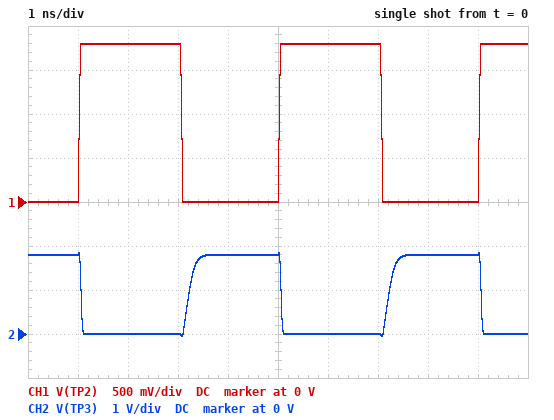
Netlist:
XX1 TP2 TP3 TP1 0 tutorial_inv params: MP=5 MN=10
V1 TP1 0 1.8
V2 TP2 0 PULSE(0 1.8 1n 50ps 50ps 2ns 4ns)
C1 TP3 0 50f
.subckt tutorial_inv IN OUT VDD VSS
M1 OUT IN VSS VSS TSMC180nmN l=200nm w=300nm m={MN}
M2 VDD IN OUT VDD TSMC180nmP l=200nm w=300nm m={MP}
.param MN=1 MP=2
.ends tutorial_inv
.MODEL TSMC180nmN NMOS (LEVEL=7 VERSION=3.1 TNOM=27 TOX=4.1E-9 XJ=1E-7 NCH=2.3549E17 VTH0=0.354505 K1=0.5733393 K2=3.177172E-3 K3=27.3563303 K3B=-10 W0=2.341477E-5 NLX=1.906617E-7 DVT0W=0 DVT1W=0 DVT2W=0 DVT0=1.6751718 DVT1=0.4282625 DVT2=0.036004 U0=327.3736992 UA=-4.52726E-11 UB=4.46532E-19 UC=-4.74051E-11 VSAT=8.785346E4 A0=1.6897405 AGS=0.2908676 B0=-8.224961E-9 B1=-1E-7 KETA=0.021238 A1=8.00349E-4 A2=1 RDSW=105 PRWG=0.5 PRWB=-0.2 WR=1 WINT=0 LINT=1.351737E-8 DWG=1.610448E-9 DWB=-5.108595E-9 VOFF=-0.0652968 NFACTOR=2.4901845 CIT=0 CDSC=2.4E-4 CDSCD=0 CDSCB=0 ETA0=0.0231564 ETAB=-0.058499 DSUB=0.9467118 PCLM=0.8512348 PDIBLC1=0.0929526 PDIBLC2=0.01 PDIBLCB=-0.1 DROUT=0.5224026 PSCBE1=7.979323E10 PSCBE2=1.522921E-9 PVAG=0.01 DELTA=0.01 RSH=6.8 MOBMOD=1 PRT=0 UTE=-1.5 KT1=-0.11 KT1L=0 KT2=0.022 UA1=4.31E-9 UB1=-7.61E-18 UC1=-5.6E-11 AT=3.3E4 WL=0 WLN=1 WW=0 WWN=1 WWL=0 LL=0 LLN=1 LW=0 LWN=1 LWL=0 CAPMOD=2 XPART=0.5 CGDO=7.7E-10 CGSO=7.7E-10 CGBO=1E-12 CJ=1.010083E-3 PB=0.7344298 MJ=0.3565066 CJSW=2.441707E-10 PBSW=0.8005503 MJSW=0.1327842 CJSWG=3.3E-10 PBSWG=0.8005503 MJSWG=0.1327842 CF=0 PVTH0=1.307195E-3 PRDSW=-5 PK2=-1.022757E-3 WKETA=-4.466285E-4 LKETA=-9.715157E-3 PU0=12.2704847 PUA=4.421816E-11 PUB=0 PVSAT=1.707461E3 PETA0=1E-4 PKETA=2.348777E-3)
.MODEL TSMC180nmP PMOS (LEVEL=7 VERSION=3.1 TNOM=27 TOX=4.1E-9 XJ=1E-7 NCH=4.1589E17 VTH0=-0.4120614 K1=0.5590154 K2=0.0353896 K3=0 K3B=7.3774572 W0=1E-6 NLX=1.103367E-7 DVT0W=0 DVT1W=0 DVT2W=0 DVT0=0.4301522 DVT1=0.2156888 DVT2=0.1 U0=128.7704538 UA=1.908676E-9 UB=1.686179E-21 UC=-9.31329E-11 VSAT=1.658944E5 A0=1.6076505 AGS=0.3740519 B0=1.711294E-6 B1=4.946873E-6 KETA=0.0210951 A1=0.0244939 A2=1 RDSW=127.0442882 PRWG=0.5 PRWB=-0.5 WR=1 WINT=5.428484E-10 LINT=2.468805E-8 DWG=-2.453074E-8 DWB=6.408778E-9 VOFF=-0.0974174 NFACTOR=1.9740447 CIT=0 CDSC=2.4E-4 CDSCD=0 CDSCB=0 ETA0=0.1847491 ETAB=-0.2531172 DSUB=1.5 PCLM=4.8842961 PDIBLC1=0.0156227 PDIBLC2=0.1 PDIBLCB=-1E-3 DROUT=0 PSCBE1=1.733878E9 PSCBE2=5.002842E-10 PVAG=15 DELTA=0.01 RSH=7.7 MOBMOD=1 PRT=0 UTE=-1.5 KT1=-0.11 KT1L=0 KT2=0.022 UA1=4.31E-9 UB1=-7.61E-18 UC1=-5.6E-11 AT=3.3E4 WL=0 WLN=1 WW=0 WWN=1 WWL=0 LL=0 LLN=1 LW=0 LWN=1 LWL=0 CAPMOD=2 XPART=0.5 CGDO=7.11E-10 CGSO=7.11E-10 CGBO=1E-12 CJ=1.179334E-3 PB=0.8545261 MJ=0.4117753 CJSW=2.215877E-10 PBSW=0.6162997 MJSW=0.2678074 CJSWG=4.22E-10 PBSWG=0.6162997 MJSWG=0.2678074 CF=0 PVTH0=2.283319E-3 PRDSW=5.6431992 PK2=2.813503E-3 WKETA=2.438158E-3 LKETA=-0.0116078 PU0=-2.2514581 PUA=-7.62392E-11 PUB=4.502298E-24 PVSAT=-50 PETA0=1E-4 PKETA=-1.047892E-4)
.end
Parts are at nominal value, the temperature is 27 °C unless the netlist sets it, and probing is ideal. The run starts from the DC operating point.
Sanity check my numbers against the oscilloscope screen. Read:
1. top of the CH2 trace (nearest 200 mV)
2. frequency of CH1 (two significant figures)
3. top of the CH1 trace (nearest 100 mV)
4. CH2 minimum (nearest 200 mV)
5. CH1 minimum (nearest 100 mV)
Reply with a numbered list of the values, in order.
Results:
1. 1.8 V
2. 250 MHz
3. 1.8 V
4. 0 V
5. 0 V
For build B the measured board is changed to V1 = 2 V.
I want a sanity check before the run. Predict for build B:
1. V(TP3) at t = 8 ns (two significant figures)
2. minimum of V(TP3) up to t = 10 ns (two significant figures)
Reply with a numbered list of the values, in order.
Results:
1. 2.0 V
2. -39 mV
